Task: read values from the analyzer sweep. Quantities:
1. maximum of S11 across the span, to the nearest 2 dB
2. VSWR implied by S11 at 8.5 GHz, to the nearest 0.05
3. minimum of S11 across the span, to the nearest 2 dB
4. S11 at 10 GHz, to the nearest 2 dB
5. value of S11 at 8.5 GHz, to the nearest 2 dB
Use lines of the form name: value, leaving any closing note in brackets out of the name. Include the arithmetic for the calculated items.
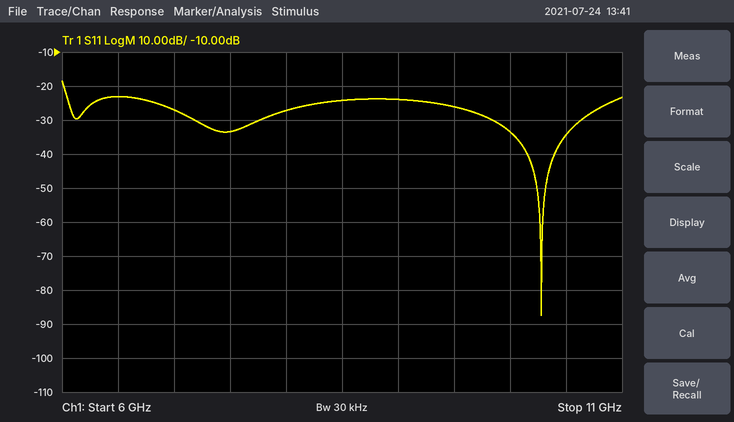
maximum of S11 across the span, to the nearest 2 dB: -18 dB
VSWR implied by S11 at 8.5 GHz, to the nearest 0.05: |Γ| = 10^(-24/20) = 0.0631; VSWR = (1 + 0.0631)/(1 − 0.0631) ≈ 1.13, so 1.15 to the nearest 0.05
minimum of S11 across the span, to the nearest 2 dB: -88 dB
S11 at 10 GHz, to the nearest 2 dB: -34 dB
value of S11 at 8.5 GHz, to the nearest 2 dB: -24 dB
